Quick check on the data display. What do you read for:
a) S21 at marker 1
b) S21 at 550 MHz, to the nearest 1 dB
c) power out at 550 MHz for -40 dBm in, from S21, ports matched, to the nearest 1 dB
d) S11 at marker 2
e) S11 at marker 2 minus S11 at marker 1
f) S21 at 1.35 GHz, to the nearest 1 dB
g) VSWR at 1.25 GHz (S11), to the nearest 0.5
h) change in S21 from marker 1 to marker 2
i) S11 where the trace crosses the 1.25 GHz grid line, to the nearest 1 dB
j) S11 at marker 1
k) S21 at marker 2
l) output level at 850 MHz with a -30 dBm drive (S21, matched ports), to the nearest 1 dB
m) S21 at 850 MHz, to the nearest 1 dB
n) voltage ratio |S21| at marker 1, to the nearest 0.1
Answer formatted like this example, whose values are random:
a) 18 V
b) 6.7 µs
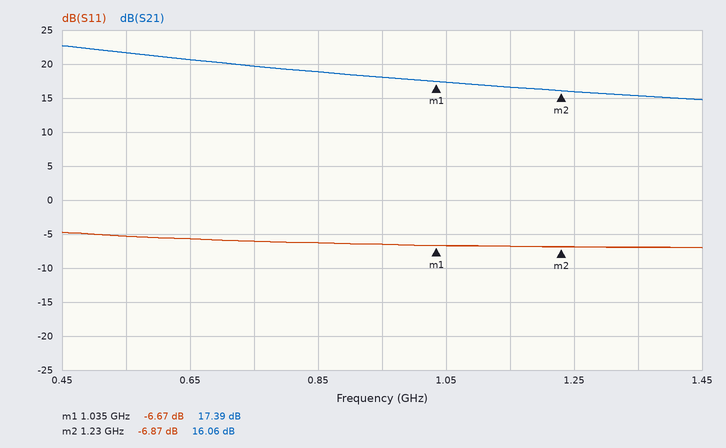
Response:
a) 17.39 dB
b) 22 dB
c) -18 dBm
d) -6.87 dB
e) -0.20 dB
f) 15 dB
g) 2.5
h) -1.33 dB
i) -7 dB
j) -6.67 dB
k) 16.06 dB
l) -11 dBm
m) 19 dB
n) 7.4
